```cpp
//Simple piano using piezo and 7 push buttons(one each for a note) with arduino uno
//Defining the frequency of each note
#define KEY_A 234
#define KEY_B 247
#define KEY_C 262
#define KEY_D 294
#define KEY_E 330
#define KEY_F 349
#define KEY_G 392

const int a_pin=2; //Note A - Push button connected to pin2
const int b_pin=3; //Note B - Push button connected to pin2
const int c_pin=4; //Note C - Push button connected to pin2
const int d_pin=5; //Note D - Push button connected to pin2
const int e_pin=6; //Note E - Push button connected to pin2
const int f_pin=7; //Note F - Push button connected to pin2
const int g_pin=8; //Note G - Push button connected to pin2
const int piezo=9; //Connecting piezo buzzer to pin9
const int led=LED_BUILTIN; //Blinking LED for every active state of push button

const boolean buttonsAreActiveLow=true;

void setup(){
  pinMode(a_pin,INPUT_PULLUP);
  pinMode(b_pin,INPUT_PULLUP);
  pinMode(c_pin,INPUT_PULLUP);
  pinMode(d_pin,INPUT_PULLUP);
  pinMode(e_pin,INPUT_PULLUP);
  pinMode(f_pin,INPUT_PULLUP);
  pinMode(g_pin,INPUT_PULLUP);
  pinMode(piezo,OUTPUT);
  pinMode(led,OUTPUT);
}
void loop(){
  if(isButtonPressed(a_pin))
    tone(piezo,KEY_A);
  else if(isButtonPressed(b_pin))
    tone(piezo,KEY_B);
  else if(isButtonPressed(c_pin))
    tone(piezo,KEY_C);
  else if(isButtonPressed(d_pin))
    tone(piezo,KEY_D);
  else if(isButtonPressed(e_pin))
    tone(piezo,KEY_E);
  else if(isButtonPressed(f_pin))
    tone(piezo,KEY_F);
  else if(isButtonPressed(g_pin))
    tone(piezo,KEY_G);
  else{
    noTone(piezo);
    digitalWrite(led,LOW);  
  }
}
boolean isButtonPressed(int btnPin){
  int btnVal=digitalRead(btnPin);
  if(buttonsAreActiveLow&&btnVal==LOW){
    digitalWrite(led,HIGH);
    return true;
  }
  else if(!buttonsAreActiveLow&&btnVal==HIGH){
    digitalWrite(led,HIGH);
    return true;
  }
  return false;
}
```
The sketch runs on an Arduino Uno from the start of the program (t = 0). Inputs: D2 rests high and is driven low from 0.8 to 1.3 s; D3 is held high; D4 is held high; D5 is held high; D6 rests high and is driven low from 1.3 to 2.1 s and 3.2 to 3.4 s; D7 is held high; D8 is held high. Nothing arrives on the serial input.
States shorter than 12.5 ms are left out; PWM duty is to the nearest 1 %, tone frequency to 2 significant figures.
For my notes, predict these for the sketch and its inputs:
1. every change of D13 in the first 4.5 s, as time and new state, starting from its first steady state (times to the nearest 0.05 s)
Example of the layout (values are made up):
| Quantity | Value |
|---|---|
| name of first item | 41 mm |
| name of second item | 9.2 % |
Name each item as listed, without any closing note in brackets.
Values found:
| Quantity | Value |
|---|---|
| every change of D13 in the first 4.5 s, as time and new state, starting from its first steady state | 0 s low; 0.8 s high; 2.1 s low; 3.2 s high; 3.4 s low |
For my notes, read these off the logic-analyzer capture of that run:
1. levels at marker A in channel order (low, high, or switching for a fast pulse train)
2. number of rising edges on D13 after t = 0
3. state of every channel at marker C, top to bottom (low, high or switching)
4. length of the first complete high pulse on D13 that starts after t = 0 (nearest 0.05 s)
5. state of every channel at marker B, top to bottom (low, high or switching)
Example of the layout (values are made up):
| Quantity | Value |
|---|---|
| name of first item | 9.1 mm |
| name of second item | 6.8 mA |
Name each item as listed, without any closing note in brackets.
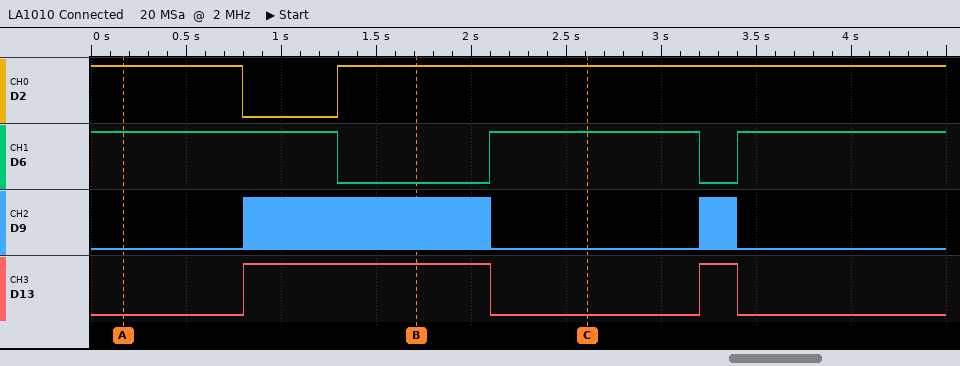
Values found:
| Quantity | Value |
|---|---|
| levels at marker A in channel order | D2 high, D6 high, D9 low, D13 low |
| number of rising edges on D13 after t = 0 | 2 |
| state of every channel at marker C, top to bottom | D2 high, D6 high, D9 low, D13 low |
| length of the first complete high pulse on D13 that starts after t = 0 | 1.30 s |
| state of every channel at marker B, top to bottom | D2 high, D6 low, D9 switching, D13 high |
